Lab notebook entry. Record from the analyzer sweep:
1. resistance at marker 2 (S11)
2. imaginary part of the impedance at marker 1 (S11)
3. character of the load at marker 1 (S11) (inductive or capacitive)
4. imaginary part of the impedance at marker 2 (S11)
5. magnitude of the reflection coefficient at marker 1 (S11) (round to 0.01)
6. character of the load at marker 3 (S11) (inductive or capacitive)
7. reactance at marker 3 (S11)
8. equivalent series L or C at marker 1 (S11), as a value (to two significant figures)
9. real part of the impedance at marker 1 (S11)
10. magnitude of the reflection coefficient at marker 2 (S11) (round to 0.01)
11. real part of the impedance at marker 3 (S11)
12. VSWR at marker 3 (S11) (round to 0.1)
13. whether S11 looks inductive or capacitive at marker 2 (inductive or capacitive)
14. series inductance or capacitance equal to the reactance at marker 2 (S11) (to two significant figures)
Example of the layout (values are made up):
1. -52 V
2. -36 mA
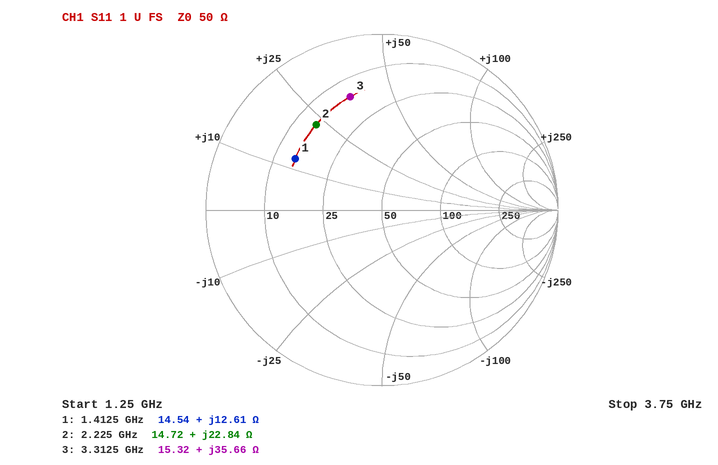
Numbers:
1. 14.72 Ω
2. +12.61 Ω
3. inductive
4. +22.84 Ω
5. 0.57
6. inductive
7. +35.66 Ω
8. 1.4 nH
9. 14.54 Ω
10. 0.61
11. 15.32 Ω
12. 5.0
13. inductive
14. 1.6 nH
